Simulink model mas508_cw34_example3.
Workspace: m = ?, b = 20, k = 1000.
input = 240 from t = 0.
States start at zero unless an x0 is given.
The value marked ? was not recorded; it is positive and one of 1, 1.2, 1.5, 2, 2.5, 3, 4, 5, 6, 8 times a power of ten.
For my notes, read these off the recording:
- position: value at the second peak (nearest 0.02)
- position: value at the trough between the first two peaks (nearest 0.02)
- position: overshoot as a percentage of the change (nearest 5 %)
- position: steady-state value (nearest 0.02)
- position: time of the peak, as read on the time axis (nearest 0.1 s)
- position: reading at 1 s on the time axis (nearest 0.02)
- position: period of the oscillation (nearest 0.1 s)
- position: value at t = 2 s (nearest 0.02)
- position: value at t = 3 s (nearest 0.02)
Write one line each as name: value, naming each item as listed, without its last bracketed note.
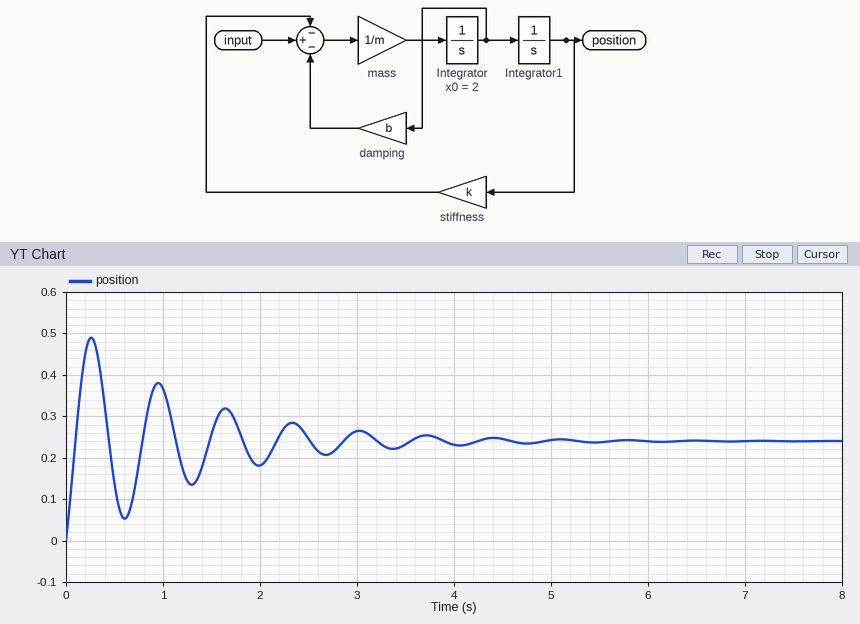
position: value at the second peak: 0.38
position: value at the trough between the first two peaks: 0.06
position: overshoot as a percentage of the change: 105 %
position: steady-state value: 0.24
position: time of the peak, as read on the time axis: 0.3 s
position: reading at 1 s on the time axis: 0.36
position: period of the oscillation: 0.7 s
position: value at t = 2 s: 0.18
position: value at t = 3 s: 0.26
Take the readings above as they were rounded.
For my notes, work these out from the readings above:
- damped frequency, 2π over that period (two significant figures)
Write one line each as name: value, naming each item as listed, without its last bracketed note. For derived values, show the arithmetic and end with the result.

damped frequency, 2π over that period: 2π / 0.7 = 9.0 rad/s
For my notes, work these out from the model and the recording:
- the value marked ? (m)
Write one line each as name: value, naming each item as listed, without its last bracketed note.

the value marked ?: 12
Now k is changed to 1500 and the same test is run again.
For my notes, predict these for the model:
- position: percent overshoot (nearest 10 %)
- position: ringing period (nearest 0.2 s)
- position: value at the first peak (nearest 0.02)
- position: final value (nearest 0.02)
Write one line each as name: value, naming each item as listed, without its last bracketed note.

position: percent overshoot: 120 %
position: ringing period: 0.6 s
position: value at the first peak: 0.36
position: final value: 0.16
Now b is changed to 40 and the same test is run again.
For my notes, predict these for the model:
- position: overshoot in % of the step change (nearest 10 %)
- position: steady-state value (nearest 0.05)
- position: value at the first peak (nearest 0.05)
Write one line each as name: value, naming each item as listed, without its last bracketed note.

position: overshoot in % of the step change: 80 %
position: steady-state value: 0.25
position: value at the first peak: 0.45
